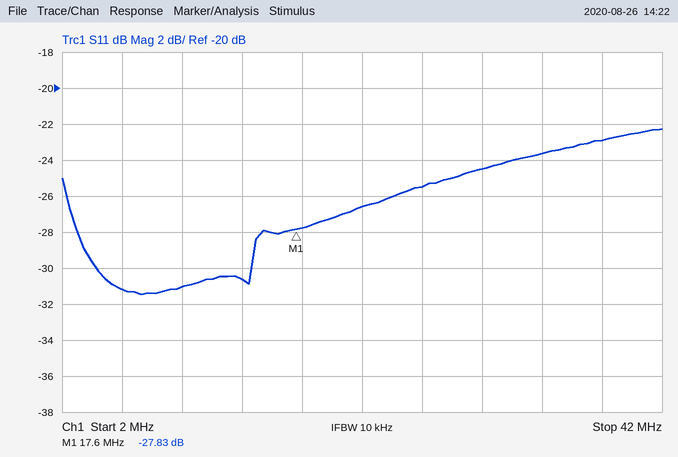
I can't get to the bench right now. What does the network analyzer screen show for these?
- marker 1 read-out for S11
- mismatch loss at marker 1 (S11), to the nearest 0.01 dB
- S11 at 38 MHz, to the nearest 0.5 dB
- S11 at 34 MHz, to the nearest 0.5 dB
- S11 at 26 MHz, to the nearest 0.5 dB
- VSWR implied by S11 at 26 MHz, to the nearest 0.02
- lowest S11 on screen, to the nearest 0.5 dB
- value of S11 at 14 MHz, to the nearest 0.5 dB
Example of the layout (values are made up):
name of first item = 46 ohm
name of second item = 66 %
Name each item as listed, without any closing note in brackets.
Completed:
marker 1 read-out for S11 = -27.83 dB
mismatch loss at marker 1 (S11), to the nearest 0.01 dB = 0.01 dB
S11 at 38 MHz, to the nearest 0.5 dB = -23.0 dB
S11 at 34 MHz, to the nearest 0.5 dB = -23.5 dB
S11 at 26 MHz, to the nearest 0.5 dB = -25.5 dB
VSWR implied by S11 at 26 MHz, to the nearest 0.02 = 1.12
lowest S11 on screen, to the nearest 0.5 dB = -31.5 dB
value of S11 at 14 MHz, to the nearest 0.5 dB = -30.5 dB
